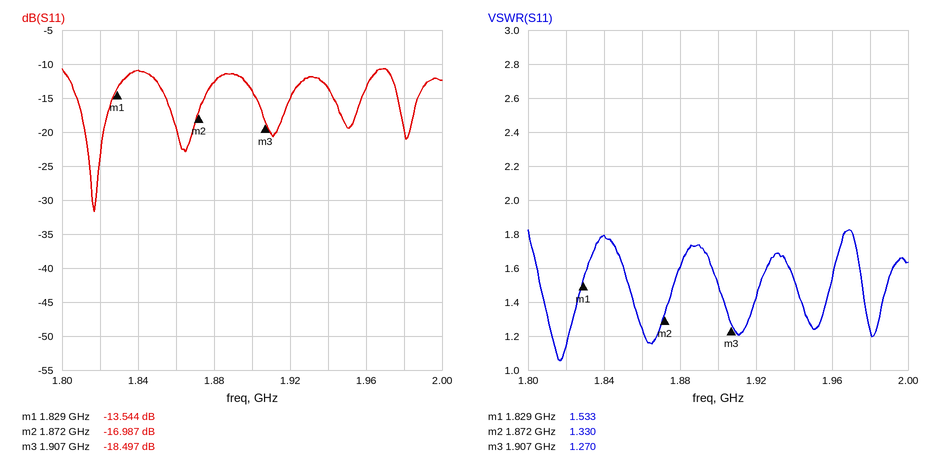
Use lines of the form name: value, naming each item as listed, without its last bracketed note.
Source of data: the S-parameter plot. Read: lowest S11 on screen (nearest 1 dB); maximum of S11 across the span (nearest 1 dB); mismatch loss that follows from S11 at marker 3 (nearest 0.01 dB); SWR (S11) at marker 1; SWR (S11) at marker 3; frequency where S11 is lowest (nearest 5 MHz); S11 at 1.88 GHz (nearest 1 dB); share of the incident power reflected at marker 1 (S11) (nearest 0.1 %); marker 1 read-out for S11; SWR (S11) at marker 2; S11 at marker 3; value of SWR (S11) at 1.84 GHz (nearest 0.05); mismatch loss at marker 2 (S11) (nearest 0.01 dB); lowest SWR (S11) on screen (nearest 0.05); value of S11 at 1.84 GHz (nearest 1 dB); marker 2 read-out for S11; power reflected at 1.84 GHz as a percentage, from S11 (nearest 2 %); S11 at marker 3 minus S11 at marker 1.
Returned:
lowest S11 on screen: -32 dB
maximum of S11 across the span: -11 dB
mismatch loss that follows from S11 at marker 3: 0.06 dB
SWR (S11) at marker 1: 1.533
SWR (S11) at marker 3: 1.270
frequency where S11 is lowest: 1.815 GHz
S11 at 1.88 GHz: -13 dB
share of the incident power reflected at marker 1 (S11): 4.4 %
marker 1 read-out for S11: -13.544 dB
SWR (S11) at marker 2: 1.330
S11 at marker 3: -18.497 dB
value of SWR (S11) at 1.84 GHz: 1.80
mismatch loss at marker 2 (S11): 0.09 dB
lowest SWR (S11) on screen: 1.05
value of S11 at 1.84 GHz: -11 dB
marker 2 read-out for S11: -16.987 dB
power reflected at 1.84 GHz as a percentage, from S11: 8 %
S11 at marker 3 minus S11 at marker 1: -4.953 dB
